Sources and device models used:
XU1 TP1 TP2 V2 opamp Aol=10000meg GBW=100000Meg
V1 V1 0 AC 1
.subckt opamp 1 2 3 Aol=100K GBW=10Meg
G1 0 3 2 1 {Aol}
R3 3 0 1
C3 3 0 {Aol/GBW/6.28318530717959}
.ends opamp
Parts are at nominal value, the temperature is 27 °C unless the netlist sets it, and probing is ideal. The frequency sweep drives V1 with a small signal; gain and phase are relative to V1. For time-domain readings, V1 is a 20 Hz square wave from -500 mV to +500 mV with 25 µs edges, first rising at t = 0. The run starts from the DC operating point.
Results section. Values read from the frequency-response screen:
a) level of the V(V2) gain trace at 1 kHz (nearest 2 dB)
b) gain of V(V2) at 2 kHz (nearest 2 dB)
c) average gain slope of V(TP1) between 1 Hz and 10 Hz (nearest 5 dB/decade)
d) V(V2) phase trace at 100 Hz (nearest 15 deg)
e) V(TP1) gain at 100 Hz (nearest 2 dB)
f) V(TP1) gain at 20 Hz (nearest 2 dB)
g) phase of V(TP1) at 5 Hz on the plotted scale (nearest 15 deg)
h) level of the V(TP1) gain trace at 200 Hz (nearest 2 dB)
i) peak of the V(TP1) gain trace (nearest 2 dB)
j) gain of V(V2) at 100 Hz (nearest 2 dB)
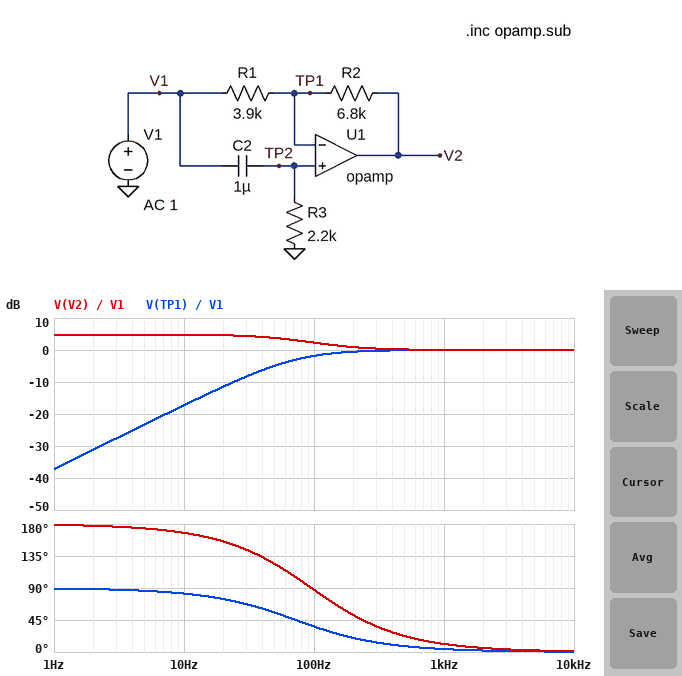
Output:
0 dB
0 dB
20 dB/decade
90 deg
-2 dB
-12 dB
90 deg
0 dB
0 dB
2 dB
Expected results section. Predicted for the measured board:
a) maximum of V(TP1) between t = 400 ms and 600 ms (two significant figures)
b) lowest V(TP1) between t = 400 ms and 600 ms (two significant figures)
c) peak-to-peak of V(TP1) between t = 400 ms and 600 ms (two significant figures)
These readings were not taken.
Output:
990 mV
-990 mV
2.0 V
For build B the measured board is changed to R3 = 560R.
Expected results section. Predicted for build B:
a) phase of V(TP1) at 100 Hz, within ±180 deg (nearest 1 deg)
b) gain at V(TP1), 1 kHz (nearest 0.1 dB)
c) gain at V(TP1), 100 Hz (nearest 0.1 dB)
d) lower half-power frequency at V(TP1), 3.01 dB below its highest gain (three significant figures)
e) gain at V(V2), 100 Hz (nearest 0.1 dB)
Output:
71 deg
-0.3 dB
-9.6 dB
284 Hz
4.5 dB
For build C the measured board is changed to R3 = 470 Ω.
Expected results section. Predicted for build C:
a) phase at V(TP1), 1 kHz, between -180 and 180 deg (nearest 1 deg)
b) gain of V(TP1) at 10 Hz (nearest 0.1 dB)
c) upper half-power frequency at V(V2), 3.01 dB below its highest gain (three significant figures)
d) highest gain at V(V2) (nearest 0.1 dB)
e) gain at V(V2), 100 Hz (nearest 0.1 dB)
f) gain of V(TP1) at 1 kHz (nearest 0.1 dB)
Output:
19 deg
-30.6 dB
579 Hz
4.8 dB
4.6 dB
-0.5 dB
